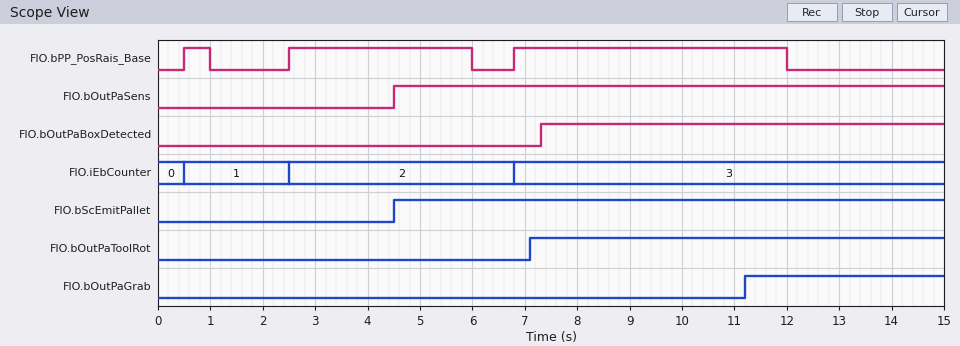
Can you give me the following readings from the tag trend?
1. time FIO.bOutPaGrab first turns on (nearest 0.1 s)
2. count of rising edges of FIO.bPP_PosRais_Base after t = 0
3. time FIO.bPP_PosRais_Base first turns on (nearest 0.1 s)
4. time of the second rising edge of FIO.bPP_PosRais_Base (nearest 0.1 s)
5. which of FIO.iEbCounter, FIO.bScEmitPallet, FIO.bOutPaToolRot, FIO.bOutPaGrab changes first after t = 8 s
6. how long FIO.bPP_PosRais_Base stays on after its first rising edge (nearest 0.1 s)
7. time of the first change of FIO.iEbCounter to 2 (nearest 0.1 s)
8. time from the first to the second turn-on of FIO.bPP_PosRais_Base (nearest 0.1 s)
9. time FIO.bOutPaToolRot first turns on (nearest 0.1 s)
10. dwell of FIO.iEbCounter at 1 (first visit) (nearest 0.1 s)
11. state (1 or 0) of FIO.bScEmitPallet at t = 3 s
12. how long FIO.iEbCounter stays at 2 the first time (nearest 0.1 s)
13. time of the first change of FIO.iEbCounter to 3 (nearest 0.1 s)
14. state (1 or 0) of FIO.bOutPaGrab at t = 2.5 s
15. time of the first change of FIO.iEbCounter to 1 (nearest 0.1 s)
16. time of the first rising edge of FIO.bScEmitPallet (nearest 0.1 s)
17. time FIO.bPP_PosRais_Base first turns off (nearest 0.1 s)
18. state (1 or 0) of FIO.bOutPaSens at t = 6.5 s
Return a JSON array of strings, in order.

["11.2 s", "3", "0.5 s", "2.5 s", "FIO.bOutPaGrab", "0.5 s", "2.5 s", "2.0 s", "7.1 s", "2.0 s", "0", "4.3 s", "6.8 s", "0", "0.5 s", "4.5 s", "1.0 s", "1"]
